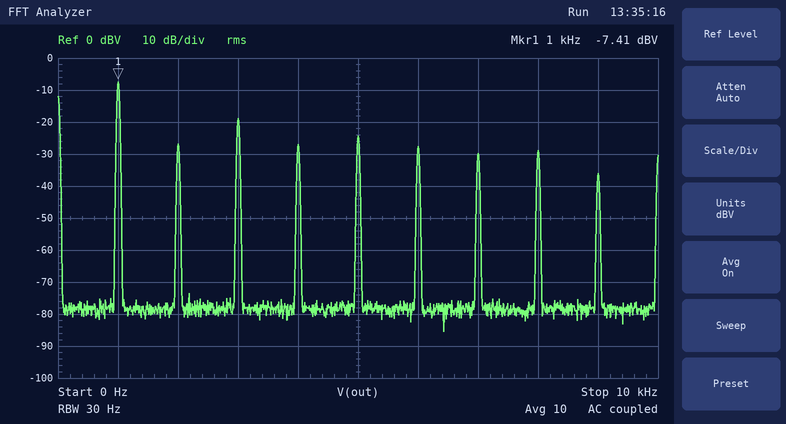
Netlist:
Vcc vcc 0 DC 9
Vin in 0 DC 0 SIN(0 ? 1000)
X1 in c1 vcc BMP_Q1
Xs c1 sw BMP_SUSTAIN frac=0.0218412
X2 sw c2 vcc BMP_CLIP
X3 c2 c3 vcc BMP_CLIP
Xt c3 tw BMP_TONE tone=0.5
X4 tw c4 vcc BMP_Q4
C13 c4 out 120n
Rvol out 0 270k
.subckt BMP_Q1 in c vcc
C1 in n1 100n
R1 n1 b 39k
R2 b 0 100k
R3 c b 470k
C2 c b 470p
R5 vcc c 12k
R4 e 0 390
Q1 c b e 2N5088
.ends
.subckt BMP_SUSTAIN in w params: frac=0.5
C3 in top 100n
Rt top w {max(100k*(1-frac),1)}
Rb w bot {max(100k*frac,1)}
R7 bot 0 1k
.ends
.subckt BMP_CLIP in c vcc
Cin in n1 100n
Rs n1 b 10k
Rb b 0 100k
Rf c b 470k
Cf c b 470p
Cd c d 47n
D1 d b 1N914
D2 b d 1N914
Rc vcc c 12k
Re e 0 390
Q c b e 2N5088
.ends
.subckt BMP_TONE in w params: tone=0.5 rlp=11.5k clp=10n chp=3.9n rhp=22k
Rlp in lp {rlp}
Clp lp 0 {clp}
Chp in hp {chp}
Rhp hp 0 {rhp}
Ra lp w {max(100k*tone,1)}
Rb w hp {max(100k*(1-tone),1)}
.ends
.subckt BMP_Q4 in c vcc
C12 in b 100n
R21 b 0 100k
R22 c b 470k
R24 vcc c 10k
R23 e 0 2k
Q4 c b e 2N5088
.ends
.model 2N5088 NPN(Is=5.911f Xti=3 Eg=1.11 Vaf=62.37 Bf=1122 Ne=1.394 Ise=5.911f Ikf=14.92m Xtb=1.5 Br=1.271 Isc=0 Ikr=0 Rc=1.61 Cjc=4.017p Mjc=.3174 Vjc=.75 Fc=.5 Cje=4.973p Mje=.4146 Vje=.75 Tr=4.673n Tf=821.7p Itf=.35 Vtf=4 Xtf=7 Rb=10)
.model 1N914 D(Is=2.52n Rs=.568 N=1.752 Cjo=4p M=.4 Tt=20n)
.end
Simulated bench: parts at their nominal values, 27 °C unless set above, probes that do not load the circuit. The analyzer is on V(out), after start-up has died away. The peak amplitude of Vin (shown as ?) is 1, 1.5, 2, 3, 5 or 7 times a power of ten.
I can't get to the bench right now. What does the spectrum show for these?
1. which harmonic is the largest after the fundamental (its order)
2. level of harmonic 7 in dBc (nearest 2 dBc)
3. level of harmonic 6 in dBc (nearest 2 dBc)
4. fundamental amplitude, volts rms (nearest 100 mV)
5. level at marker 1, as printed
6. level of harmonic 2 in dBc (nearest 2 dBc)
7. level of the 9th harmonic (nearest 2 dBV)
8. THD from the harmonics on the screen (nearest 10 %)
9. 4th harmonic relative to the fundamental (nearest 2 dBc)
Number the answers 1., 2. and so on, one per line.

1. 3
2. -22 dBc
3. -20 dBc
4. 400 mV
5. -7.41 dBV
6. -20 dBc
7. -36 dBV
8. 40 %
9. -20 dBc
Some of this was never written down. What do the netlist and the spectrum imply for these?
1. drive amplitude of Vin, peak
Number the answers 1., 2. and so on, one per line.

1. 2 V
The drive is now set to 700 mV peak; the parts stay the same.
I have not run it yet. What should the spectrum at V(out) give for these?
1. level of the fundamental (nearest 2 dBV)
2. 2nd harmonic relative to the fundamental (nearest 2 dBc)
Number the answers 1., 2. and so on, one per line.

1. -8 dBV
2. -44 dBc
